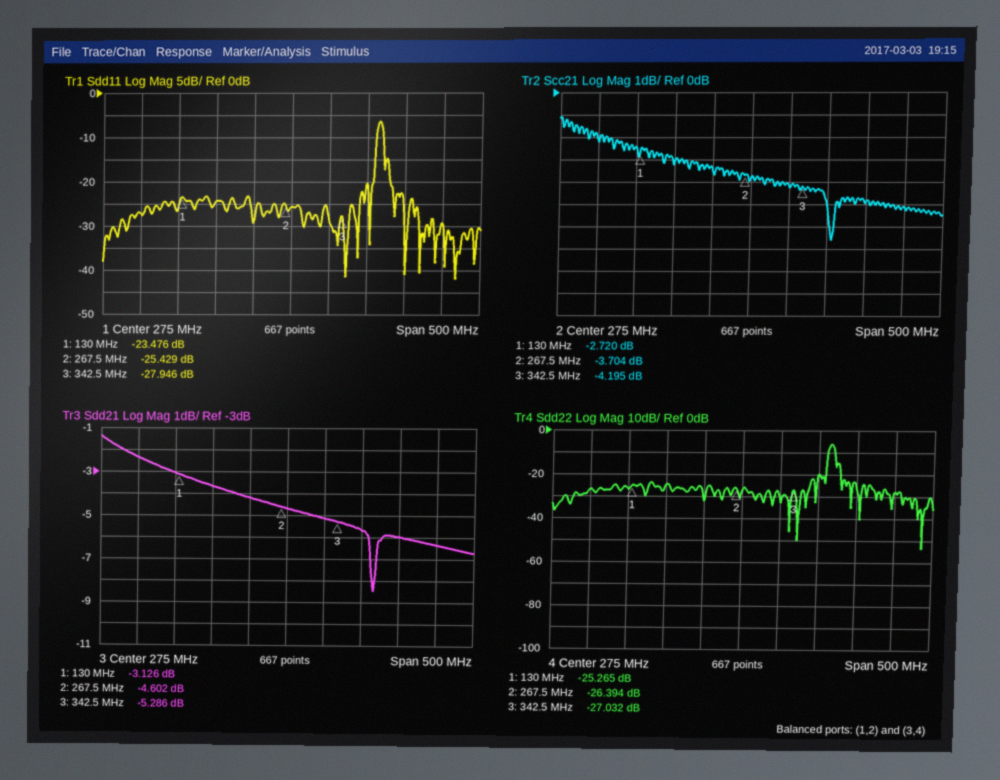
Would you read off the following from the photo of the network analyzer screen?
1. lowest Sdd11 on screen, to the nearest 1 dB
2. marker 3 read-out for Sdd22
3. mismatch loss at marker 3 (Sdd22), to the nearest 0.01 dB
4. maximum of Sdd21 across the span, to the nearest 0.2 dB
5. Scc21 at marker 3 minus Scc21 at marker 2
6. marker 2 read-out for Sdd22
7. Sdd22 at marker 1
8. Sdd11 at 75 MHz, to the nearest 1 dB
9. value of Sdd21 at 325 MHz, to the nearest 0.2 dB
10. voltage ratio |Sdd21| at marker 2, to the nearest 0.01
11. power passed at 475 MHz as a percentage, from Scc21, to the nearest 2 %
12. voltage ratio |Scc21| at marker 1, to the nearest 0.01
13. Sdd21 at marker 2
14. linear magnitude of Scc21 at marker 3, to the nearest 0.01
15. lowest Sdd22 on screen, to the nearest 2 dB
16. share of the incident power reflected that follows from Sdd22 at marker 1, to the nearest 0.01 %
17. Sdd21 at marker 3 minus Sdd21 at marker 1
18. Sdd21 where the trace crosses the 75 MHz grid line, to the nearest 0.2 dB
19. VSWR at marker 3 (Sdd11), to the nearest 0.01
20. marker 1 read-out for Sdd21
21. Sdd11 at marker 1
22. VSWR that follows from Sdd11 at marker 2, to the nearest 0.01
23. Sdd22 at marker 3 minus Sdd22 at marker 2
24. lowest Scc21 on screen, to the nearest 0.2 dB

-42 dB
-27.032 dB
0.01 dB
-1.4 dB
-0.491 dB
-26.394 dB
-25.265 dB
-27 dB
-5.2 dB
0.59
30 %
0.73
-4.602 dB
0.62
-54 dB
0.30 %
-2.160 dB
-2.4 dB
1.08
-3.126 dB
-23.476 dB
1.11
-0.638 dB
-6.6 dB
